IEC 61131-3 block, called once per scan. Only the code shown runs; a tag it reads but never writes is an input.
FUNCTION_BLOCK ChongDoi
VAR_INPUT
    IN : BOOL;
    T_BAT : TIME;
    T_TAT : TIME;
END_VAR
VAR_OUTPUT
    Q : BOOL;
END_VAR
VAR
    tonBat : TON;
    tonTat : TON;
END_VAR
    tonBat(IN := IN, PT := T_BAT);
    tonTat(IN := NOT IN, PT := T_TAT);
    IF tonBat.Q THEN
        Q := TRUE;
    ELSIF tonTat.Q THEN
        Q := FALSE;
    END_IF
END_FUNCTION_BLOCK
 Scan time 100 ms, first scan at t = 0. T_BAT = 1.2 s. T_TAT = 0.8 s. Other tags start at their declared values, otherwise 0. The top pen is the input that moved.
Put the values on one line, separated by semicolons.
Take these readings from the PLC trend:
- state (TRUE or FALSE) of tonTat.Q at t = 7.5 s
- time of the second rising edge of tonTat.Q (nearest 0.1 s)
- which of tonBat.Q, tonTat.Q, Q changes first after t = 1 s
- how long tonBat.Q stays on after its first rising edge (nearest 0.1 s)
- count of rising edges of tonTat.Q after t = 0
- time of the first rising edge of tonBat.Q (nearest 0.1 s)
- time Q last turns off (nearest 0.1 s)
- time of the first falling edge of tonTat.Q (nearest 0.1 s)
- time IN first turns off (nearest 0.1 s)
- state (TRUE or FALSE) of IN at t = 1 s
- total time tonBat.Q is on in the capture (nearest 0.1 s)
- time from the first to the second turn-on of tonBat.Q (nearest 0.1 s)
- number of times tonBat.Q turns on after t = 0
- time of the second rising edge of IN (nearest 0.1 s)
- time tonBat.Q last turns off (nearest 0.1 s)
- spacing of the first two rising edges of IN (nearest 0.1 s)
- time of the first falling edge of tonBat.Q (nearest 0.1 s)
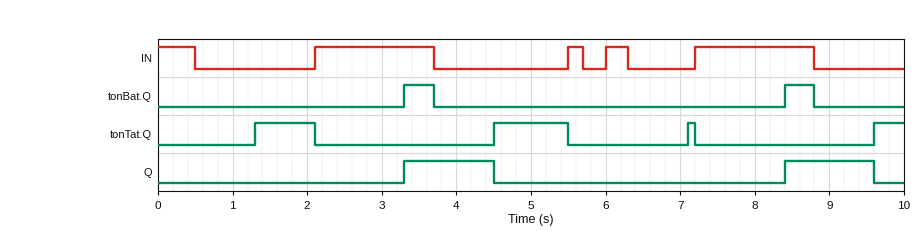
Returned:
FALSE; 4.5 s; tonTat.Q; 0.4 s; 4; 3.3 s; 9.6 s; 2.1 s; 0.5 s; FALSE; 0.8 s; 5.1 s; 2; 5.5 s; 8.8 s; 3.4 s; 3.7 s
